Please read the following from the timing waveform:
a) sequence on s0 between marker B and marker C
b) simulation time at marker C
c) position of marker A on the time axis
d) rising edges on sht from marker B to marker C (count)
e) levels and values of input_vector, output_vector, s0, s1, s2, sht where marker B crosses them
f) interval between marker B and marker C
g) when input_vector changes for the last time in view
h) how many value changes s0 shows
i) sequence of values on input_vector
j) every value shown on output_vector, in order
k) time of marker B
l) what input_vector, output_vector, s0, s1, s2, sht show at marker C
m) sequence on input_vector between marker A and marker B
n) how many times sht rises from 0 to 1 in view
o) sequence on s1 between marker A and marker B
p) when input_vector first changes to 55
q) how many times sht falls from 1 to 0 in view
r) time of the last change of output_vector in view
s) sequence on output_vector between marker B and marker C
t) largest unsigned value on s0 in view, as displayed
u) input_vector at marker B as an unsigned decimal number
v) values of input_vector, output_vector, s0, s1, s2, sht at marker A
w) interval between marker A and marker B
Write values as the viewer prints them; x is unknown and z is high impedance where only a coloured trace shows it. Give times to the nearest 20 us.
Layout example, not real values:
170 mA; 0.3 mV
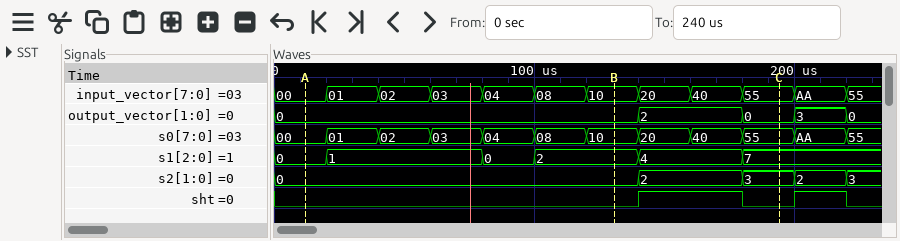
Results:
10, 20, 40, 55; 200 us; 20 us; 1; input_vector=10, output_vector=0, s0=10, s1=2, s2=0, sht=0; 60 us; 220 us; 11; 00, 01, 02, 03, 04, 08, 10, 20, 40, 55, AA, 55; 0, 2, 0, 3, 0; 140 us; input_vector=55, output_vector=0, s0=55, s1=7, s2=3, sht=0; 00, 01, 02, 03, 04, 08, 10; 2; 0, 1, 0, 2; 180 us; 2; 220 us; 0, 2, 0; AA; 16; input_vector=00, output_vector=0, s0=00, s1=0, s2=0, sht=0; 120 us
